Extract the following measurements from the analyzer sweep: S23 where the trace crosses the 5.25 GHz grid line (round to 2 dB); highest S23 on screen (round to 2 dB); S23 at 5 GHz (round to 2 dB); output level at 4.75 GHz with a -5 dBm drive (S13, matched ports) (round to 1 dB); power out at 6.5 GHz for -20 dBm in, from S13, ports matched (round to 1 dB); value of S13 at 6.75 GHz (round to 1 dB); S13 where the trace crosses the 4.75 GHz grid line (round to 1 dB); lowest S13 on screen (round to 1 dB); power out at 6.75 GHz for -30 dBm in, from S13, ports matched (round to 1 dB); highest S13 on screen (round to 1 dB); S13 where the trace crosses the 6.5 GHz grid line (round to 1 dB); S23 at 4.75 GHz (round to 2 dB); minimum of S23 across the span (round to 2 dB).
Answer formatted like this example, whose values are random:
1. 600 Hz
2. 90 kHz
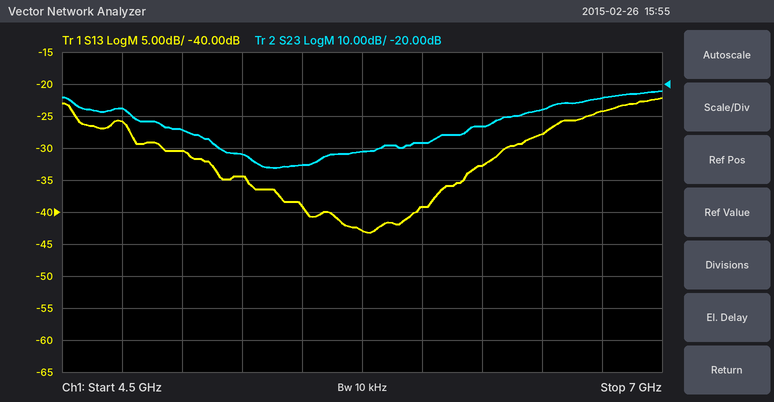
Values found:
1. -42 dB
2. -22 dB
3. -34 dB
4. -31 dBm
5. -48 dBm
6. -24 dB
7. -26 dB
8. -43 dB
9. -54 dBm
10. -22 dB
11. -28 dB
12. -28 dB
13. -46 dB
